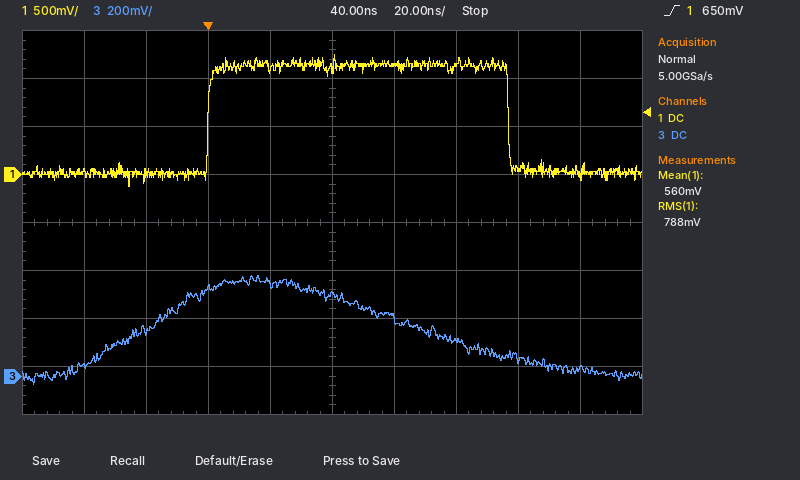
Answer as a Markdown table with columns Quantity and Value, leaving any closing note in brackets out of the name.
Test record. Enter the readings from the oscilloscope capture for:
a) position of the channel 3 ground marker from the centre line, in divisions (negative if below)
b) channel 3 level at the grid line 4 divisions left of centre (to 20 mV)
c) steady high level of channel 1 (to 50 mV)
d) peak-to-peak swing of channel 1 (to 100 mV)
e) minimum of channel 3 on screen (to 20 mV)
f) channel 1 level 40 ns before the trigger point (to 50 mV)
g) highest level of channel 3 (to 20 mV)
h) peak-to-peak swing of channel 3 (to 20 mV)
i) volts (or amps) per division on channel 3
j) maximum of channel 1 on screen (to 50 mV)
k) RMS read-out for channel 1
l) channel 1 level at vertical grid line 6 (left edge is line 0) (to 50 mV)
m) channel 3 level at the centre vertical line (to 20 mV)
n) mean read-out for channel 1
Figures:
| Quantity | Value |
|---|---|
| position of the channel 3 ground marker from the centre line, in divisions | -3.2 div |
| channel 3 level at the grid line 4 divisions left of centre | 40 mV |
| steady high level of channel 1 | 1.15 V |
| peak-to-peak swing of channel 1 | 1.40 V |
| minimum of channel 3 on screen | -40 mV |
| channel 1 level 40 ns before the trigger point | 0 mV |
| highest level of channel 3 | 420 mV |
| peak-to-peak swing of channel 3 | 460 mV |
| volts (or amps) per division on channel 3 | 200 mV |
| maximum of channel 1 on screen | 1.25 V |
| RMS read-out for channel 1 | 788 mV |
| channel 1 level at vertical grid line 6 (left edge is line 0) | 1.15 V |
| channel 3 level at the centre vertical line | 340 mV |
| mean read-out for channel 1 | 560 mV |
